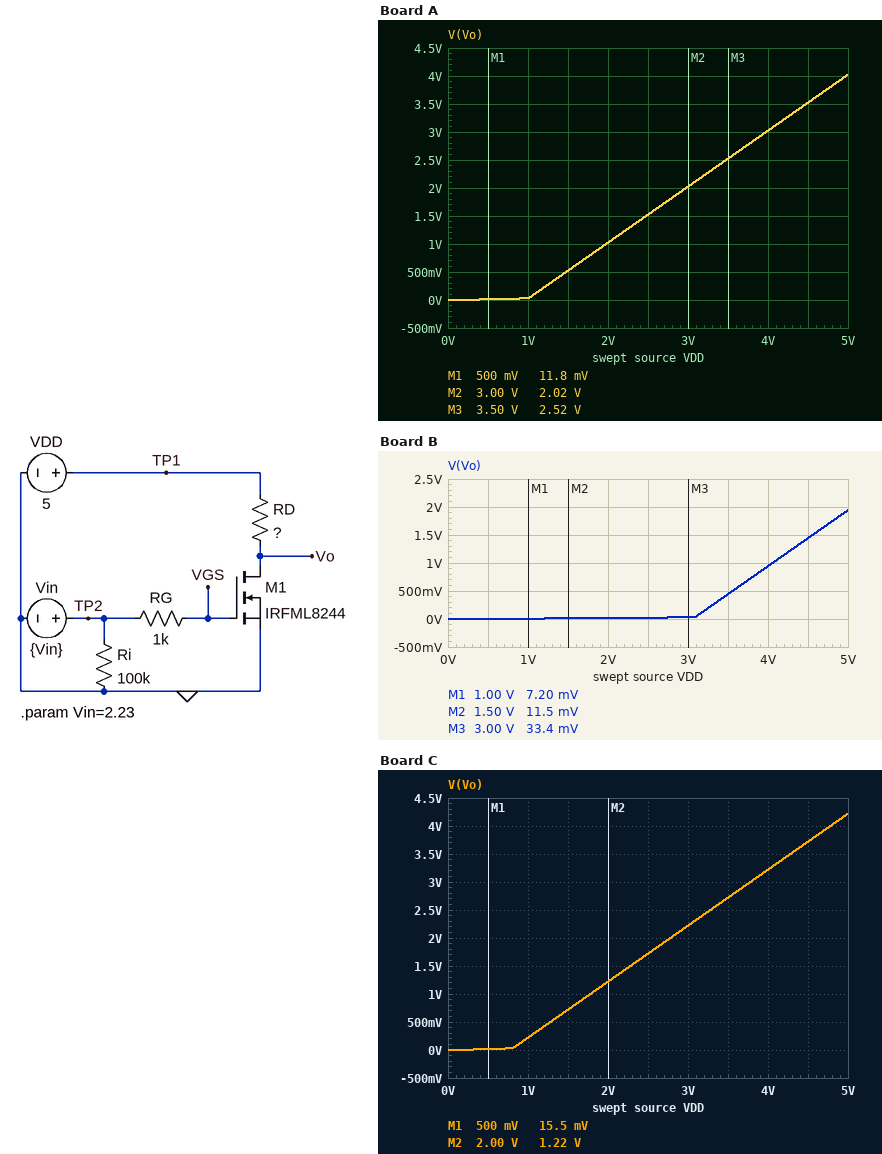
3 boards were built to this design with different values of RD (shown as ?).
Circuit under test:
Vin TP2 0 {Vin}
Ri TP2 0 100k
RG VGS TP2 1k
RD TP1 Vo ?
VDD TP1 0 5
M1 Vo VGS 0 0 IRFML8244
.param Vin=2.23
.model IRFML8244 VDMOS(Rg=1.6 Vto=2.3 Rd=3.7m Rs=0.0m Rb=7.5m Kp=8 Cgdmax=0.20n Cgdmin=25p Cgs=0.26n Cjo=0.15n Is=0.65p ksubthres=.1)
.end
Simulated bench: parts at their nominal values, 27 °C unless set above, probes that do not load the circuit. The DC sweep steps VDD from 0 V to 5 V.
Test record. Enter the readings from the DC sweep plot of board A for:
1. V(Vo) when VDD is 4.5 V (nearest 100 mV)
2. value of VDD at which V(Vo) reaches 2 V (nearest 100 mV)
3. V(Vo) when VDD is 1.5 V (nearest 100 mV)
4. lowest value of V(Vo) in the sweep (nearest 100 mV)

3.5 V
3.0 V
500 mV
0 V
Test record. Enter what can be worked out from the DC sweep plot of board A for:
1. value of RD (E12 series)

150 Ω
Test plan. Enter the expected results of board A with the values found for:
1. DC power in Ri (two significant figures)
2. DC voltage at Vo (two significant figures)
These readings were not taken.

50 µW
4.0 V
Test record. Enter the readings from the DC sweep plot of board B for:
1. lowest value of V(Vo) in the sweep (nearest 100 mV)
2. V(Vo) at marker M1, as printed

0 V
7.20 mV
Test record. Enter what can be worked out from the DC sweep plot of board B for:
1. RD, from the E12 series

470 Ω
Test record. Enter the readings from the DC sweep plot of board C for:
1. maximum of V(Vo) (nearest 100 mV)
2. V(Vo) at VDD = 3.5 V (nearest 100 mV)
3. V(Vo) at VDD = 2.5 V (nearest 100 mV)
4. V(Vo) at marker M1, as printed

4.2 V
2.7 V
1.7 V
15.5 mV
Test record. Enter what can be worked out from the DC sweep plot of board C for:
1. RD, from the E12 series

120 Ω
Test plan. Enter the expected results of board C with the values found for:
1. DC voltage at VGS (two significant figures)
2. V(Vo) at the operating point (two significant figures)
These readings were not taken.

2.2 V
4.2 V
